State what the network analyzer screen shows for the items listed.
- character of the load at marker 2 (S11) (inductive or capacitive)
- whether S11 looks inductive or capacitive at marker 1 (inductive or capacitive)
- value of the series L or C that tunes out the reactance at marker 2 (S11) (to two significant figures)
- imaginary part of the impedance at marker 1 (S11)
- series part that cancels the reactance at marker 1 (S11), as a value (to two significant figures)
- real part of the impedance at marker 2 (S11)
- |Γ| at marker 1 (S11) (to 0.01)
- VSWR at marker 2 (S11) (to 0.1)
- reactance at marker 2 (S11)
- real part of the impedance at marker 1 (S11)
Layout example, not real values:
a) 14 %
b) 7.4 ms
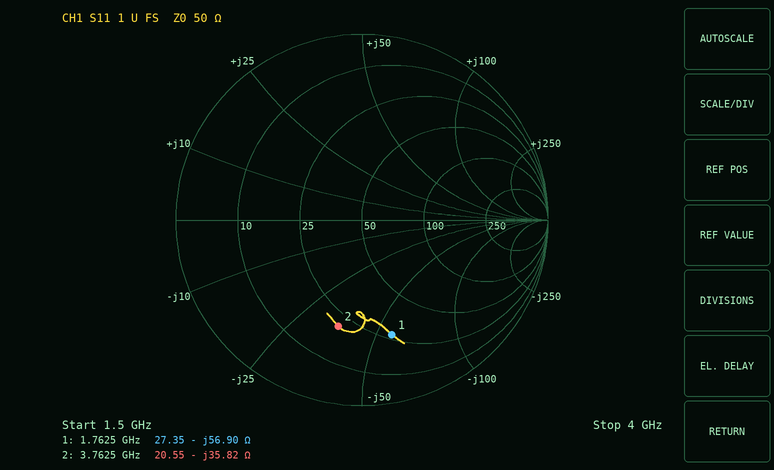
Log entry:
a) capacitive
b) capacitive
c) 1.5 nH
d) -56.90 Ω
e) 5.1 nH
f) 20.55 Ω
g) 0.64
h) 3.8
i) -35.82 Ω
j) 27.35 Ω
